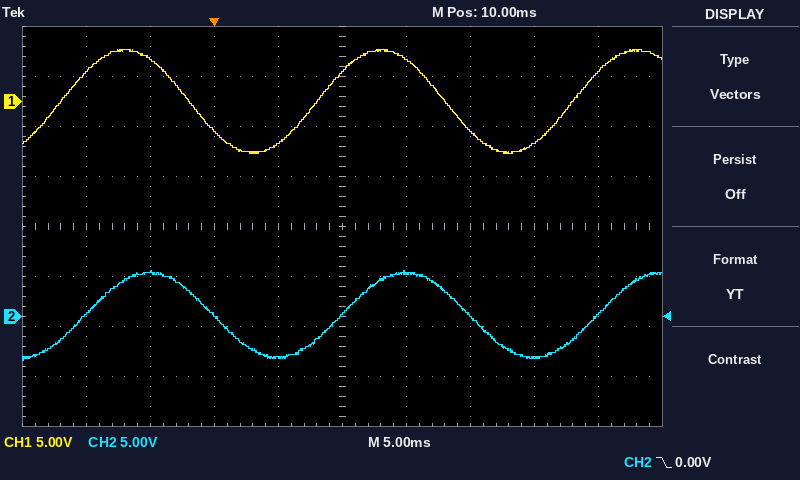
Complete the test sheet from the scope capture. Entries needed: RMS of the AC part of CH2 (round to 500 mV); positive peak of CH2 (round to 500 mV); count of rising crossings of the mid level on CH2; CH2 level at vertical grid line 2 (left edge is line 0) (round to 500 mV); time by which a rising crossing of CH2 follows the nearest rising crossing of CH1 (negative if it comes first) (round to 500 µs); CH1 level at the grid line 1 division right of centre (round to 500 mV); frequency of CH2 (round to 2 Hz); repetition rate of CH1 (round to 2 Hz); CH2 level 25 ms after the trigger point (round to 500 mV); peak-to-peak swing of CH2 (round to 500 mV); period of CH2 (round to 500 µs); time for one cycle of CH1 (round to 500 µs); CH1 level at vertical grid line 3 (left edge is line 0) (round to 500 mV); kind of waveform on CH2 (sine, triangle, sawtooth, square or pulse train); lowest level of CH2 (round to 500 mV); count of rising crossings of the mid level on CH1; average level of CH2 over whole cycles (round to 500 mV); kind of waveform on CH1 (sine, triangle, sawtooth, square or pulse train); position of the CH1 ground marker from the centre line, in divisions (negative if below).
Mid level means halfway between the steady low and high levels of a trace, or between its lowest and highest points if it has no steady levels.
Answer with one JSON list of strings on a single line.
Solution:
["3.0 V", "4.5 V", "3", "4.5 V", "+2.0 ms", "4.0 V", "50 Hz", "50 Hz", "-4.0 V", "9.0 V", "20.0 ms", "20.0 ms", "-3.0 V", "sine", "-4.5 V", "3", "0.0 V", "sine", "+2.5 div"]
